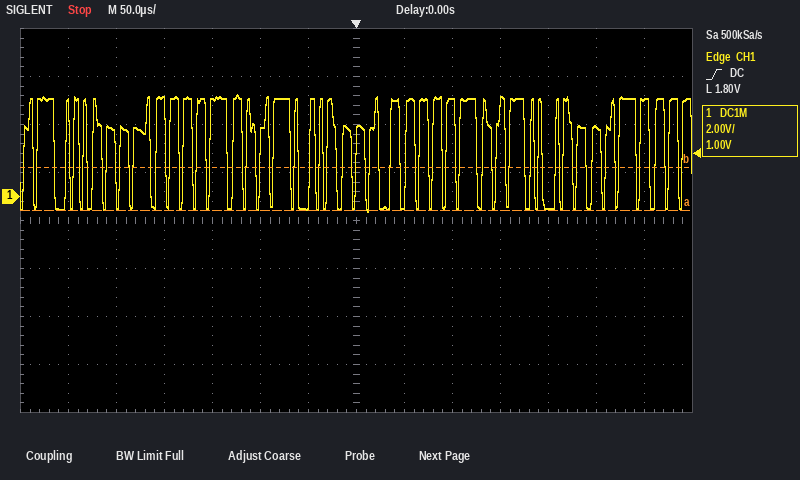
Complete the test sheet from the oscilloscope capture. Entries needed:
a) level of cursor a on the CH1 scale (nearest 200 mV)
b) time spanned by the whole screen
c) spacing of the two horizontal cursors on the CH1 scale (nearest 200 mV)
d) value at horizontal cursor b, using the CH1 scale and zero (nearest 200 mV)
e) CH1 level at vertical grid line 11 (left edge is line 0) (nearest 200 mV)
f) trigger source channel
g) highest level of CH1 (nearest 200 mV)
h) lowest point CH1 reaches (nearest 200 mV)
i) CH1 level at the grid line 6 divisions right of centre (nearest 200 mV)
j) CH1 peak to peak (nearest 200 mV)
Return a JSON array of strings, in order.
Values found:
["-600 mV", "700 µs", "1.8 V", "1.2 V", "-400 mV", "CH1", "4.2 V", "-600 mV", "4.0 V", "4.8 V"]
